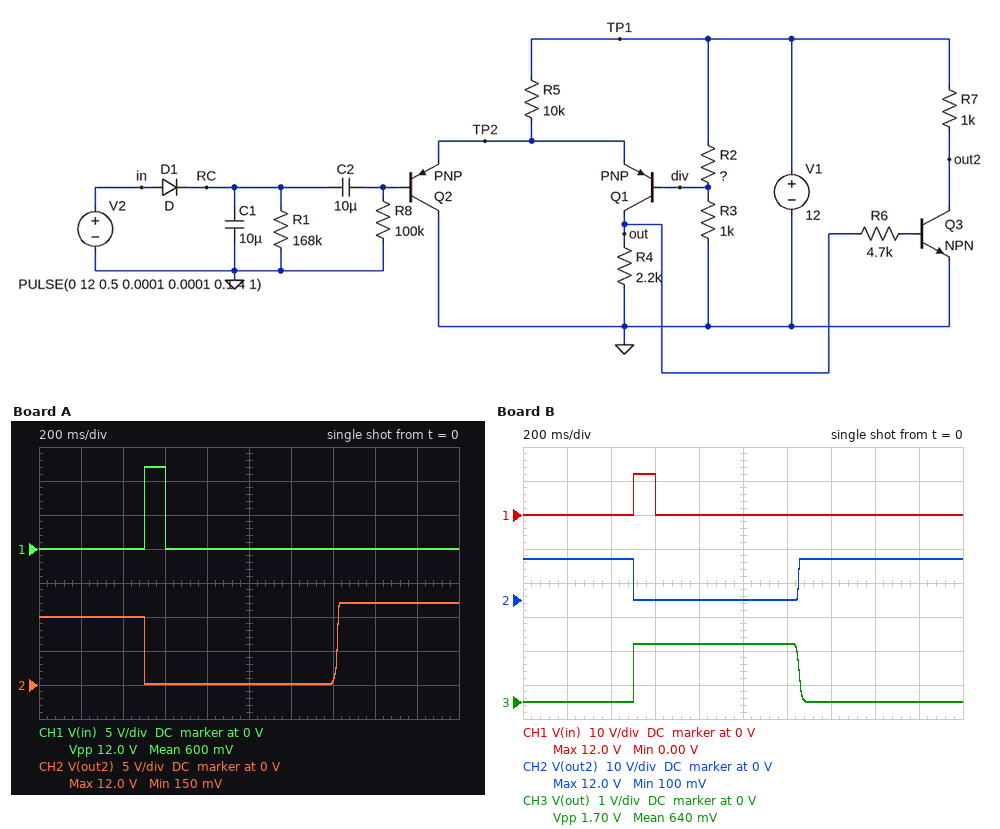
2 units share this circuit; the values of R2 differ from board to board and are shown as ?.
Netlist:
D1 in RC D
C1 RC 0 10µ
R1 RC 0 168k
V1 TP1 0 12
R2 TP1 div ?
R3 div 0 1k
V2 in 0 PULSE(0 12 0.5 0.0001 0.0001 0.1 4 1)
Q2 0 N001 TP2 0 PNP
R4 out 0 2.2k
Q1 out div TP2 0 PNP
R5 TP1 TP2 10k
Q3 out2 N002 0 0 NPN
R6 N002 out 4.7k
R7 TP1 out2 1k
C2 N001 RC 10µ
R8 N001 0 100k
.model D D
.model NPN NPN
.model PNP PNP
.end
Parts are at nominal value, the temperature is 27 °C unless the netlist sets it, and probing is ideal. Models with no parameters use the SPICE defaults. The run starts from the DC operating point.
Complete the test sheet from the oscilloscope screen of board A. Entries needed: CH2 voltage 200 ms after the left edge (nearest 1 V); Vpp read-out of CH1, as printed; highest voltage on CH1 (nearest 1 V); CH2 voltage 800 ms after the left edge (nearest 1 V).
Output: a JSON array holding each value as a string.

["10 V", "12.0 V", "12 V", "0 V"]
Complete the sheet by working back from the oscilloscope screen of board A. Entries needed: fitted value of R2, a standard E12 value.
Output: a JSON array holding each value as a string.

["18 kΩ"]
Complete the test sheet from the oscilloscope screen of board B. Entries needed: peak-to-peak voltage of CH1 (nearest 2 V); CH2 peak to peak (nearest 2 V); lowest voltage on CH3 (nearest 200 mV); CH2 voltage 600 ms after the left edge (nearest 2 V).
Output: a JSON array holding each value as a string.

["12 V", "12 V", "0 V", "0 V"]
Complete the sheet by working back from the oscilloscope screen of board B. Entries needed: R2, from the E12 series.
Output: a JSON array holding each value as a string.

["6.8 kΩ"]
